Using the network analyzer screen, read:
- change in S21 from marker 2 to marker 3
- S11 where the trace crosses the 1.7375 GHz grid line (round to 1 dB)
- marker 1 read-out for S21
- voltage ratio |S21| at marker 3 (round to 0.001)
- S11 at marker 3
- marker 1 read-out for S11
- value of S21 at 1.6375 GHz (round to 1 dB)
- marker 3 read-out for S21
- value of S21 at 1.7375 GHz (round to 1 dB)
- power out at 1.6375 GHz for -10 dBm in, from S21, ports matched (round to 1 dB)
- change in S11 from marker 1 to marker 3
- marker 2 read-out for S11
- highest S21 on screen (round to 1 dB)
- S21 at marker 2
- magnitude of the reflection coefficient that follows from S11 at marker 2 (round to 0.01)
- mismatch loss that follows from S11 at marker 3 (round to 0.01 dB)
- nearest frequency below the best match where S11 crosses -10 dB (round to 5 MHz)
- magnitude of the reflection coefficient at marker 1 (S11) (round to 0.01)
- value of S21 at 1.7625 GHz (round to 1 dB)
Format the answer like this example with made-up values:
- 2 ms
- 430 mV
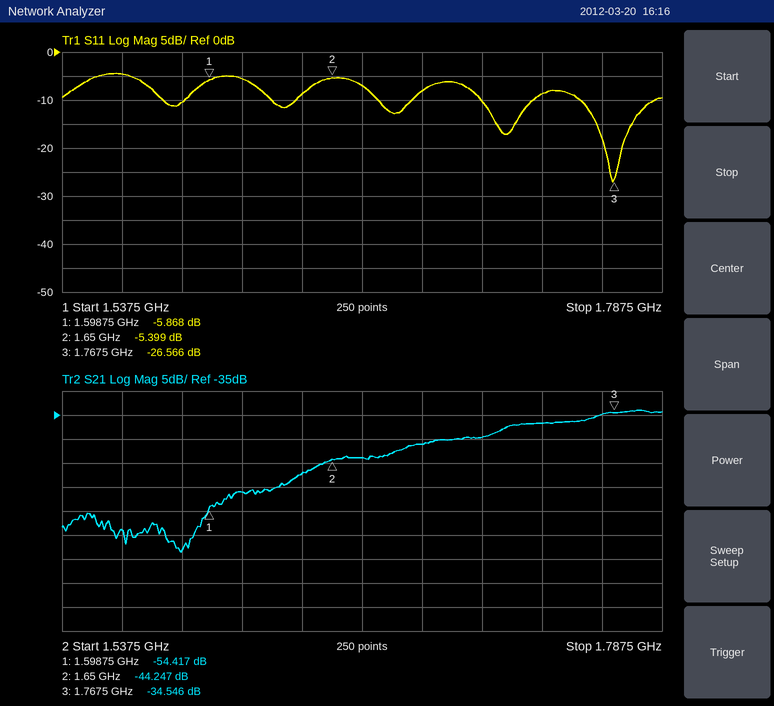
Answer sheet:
- 9.701 dB
- -9 dB
- -54.417 dB
- 0.019
- -26.566 dB
- -5.868 dB
- -47 dB
- -34.546 dB
- -37 dB
- -57 dBm
- -20.698 dB
- -5.399 dB
- -34 dB
- -44.247 dB
- 0.54
- 0.01 dB
- 1.755 GHz
- 0.51
- -35 dB
